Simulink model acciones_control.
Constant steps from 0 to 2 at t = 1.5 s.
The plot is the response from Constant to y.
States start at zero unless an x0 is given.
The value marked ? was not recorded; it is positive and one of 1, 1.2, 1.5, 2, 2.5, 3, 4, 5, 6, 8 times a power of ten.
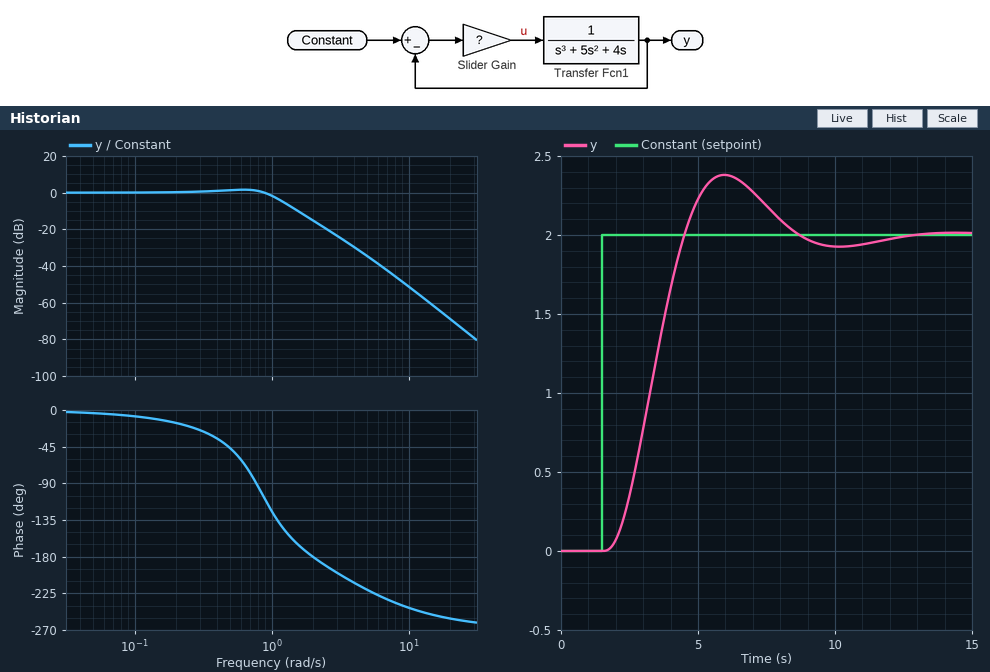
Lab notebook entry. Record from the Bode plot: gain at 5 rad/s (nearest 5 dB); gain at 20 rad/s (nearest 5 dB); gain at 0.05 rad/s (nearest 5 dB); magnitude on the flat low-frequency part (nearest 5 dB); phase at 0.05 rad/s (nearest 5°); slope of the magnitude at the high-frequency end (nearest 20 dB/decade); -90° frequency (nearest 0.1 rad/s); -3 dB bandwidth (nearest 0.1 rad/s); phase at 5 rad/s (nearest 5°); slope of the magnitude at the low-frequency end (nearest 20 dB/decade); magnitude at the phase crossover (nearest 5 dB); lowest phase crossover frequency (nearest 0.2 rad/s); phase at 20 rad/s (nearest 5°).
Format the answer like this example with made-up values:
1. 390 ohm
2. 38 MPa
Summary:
1. -35 dB
2. -70 dB
3. 0 dB
4. 0 dB
5. -5°
6. -60 dB/decade
7. 0.8 rad/s
8. 1.1 rad/s
9. -220°
10. 0 dB/decade
11. -15 dB
12. 2.0 rad/s
13. -255°
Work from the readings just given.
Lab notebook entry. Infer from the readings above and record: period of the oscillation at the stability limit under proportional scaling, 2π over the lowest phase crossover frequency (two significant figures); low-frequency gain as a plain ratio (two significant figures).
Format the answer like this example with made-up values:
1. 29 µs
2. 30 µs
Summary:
1. 3.1 s
2. 1.0
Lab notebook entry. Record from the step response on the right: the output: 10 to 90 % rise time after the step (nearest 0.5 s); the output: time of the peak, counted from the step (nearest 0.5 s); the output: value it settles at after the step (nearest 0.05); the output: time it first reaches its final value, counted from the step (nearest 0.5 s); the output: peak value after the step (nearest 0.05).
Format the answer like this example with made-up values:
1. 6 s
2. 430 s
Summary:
1. 2.0 s
2. 4.5 s
3. 2.00
4. 3.0 s
5. 2.40
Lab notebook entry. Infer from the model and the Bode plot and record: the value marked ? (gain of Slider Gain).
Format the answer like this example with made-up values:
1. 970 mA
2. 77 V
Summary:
1. 3
